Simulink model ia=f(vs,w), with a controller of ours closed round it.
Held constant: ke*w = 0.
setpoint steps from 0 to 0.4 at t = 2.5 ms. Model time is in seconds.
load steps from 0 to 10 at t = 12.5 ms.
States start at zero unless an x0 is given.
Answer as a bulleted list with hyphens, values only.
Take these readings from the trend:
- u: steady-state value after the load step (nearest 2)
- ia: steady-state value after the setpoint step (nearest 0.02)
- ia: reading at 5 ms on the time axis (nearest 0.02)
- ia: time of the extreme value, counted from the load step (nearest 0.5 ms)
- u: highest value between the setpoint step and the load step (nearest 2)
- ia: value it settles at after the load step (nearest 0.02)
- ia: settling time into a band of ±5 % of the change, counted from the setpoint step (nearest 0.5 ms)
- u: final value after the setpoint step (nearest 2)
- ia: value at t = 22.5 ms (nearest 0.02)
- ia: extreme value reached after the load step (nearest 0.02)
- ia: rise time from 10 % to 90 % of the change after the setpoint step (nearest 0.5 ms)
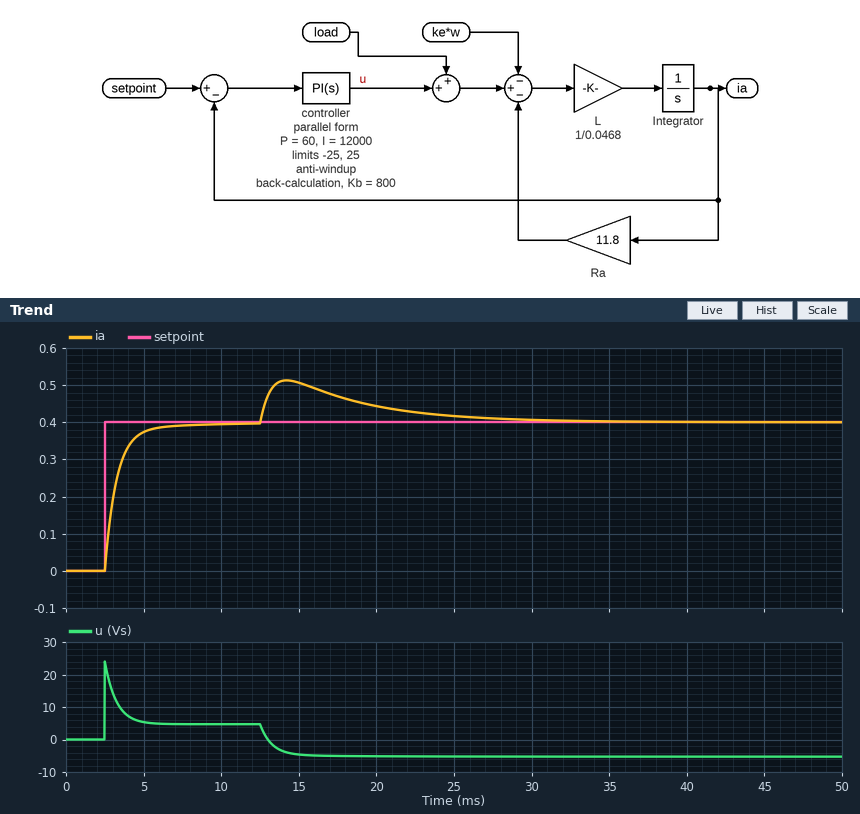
- -6
- 0.40
- 0.38
- 1.5 ms
- 24
- 0.40
- 3.0 ms
- 4
- 0.42
- 0.52
- 2.0 ms
